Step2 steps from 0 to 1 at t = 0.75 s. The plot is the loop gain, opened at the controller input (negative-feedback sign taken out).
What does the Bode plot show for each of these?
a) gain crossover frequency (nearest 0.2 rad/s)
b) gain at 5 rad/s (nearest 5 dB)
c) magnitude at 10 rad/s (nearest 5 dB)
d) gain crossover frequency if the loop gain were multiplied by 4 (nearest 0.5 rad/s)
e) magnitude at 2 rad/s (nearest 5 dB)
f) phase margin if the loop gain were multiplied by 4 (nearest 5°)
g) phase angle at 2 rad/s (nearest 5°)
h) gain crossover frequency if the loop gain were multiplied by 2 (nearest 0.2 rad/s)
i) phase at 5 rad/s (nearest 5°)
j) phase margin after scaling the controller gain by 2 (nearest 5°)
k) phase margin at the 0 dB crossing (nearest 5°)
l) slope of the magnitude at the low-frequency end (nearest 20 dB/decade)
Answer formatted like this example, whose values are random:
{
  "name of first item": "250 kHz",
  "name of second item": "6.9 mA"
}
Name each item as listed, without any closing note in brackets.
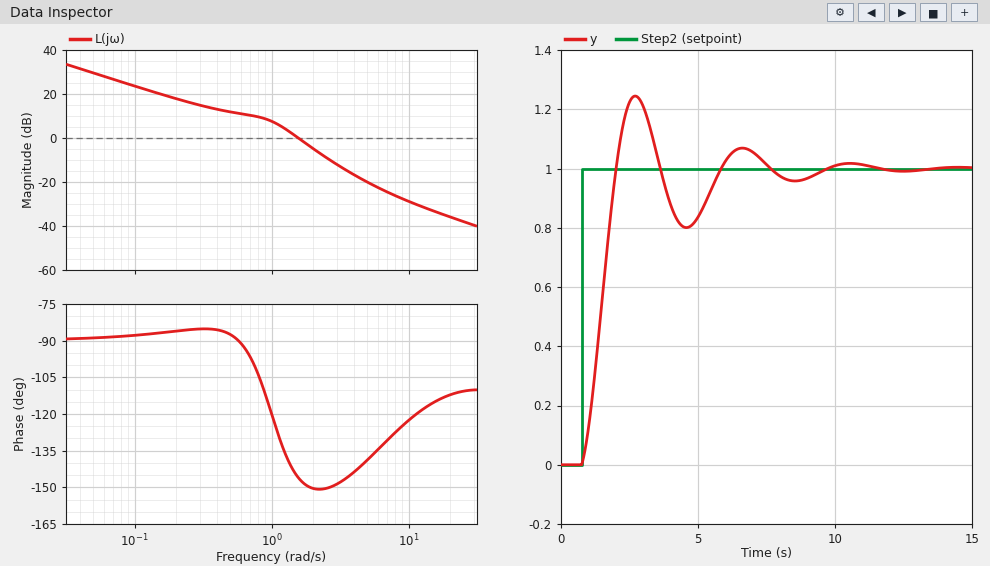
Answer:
{
  "gain crossover frequency": "1.6 rad/s",
  "gain at 5 rad/s": "-20 dB",
  "magnitude at 10 rad/s": "-30 dB",
  "gain crossover frequency if the loop gain were multiplied by 4": "3.0 rad/s",
  "magnitude at 2 rad/s": "-5 dB",
  "phase margin if the loop gain were multiplied by 4": "30°",
  "phase angle at 2 rad/s": "-150°",
  "gain crossover frequency if the loop gain were multiplied by 2": "2.2 rad/s",
  "phase at 5 rad/s": "-140°",
  "phase margin after scaling the controller gain by 2": "30°",
  "phase margin at the 0 dB crossing": "35°",
  "slope of the magnitude at the low-frequency end": "-20 dB/decade"
}
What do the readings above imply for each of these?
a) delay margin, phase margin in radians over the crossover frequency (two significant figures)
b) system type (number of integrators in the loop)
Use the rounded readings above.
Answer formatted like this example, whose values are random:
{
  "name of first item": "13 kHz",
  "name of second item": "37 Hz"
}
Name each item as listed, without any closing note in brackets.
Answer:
{
  "delay margin, phase margin in radians over the crossover frequency": "0.38 s",
  "system type": "1"
}
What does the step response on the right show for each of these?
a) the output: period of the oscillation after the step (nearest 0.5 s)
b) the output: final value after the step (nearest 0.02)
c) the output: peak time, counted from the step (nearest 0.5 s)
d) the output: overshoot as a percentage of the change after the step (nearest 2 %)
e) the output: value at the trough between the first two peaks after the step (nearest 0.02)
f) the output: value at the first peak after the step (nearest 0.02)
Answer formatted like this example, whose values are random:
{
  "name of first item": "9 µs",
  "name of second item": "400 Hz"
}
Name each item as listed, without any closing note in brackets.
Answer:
{
  "the output: period of the oscillation after the step": "4.0 s",
  "the output: final value after the step": "1.00",
  "the output: peak time, counted from the step": "2.0 s",
  "the output: overshoot as a percentage of the change after the step": "24 %",
  "the output: value at the trough between the first two peaks after the step": "0.80",
  "the output: value at the first peak after the step": "1.24"
}
